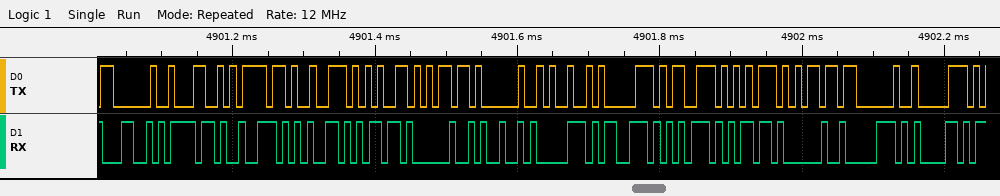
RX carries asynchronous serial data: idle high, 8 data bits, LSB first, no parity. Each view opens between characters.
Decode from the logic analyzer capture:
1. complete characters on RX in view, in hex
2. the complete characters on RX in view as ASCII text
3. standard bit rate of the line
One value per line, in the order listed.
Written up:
4C, 6F, 72, 65, 6D, 20, 49, 70, 73, 75, 6D, 20, 70, 61
"Lorem Ipsum pa"
115200 baud
